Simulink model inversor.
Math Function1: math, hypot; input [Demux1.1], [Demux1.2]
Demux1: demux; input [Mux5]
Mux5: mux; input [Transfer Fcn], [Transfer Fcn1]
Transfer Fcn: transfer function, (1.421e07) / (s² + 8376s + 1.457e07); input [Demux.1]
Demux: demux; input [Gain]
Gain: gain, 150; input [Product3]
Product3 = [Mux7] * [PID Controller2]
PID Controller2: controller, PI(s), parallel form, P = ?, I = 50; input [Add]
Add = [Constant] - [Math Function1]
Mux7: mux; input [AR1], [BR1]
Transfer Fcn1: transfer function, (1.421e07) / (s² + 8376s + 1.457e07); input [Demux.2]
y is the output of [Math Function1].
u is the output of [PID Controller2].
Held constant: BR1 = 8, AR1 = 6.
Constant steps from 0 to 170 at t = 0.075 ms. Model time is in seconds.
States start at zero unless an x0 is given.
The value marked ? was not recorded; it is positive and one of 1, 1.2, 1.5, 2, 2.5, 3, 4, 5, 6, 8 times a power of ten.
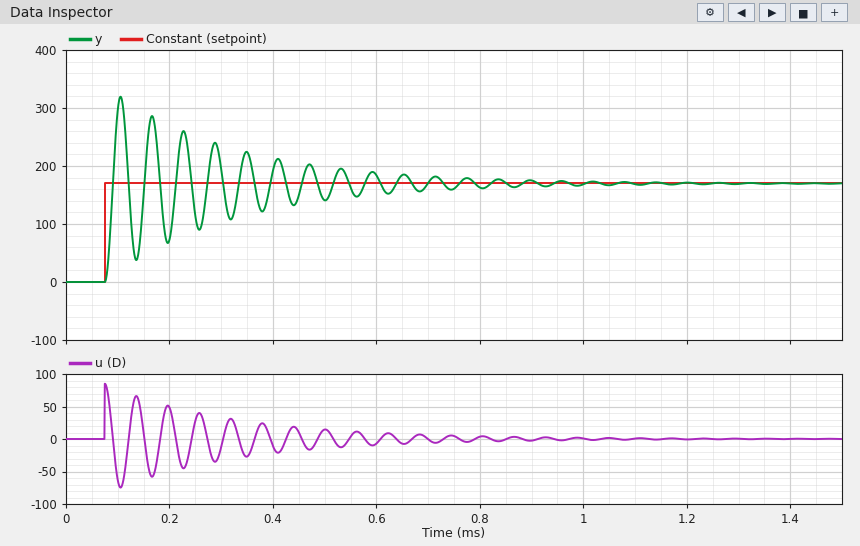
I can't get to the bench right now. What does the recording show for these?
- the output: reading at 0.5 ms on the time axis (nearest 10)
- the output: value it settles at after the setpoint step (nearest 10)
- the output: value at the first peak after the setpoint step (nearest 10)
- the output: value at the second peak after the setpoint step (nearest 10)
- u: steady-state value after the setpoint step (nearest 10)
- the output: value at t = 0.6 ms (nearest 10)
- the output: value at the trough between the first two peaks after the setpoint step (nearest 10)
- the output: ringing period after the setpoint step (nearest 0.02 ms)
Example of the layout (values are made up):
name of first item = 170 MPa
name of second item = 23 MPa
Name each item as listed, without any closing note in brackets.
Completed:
the output: reading at 0.5 ms on the time axis = 140
the output: value it settles at after the setpoint step = 170
the output: value at the first peak after the setpoint step = 320
the output: value at the second peak after the setpoint step = 290
u: steady-state value after the setpoint step = 0
the output: value at t = 0.6 ms = 180
the output: value at the trough between the first two peaks after the setpoint step = 40
the output: ringing period after the setpoint step = 0.06 ms
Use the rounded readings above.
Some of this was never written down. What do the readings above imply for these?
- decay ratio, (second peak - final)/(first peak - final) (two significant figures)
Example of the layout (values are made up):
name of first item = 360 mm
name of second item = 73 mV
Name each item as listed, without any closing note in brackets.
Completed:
decay ratio, (second peak - final)/(first peak - final) = 0.80
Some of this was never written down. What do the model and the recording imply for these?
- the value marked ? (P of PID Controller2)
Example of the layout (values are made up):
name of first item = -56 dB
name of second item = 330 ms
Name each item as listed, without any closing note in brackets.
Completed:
the value marked ? = 0.5
